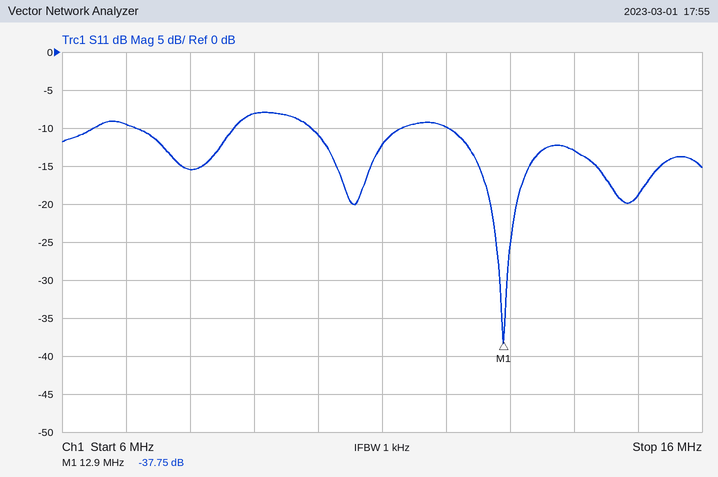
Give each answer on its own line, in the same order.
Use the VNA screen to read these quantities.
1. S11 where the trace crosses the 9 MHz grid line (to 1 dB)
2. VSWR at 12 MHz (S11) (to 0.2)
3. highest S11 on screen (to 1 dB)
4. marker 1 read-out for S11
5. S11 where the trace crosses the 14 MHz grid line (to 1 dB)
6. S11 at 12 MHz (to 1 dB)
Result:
-8 dB
2.0
-8 dB
-37.75 dB
-13 dB
-10 dB
